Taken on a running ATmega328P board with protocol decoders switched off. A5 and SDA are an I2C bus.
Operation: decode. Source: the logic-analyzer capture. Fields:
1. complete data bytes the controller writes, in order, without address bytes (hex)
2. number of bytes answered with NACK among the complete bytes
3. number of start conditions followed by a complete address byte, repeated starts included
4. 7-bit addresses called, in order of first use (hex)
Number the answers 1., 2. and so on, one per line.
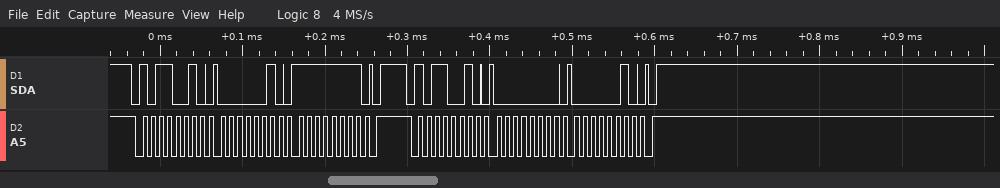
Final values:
1. 02 FF 00 02
2. 0
3. 2
4. 0x59
